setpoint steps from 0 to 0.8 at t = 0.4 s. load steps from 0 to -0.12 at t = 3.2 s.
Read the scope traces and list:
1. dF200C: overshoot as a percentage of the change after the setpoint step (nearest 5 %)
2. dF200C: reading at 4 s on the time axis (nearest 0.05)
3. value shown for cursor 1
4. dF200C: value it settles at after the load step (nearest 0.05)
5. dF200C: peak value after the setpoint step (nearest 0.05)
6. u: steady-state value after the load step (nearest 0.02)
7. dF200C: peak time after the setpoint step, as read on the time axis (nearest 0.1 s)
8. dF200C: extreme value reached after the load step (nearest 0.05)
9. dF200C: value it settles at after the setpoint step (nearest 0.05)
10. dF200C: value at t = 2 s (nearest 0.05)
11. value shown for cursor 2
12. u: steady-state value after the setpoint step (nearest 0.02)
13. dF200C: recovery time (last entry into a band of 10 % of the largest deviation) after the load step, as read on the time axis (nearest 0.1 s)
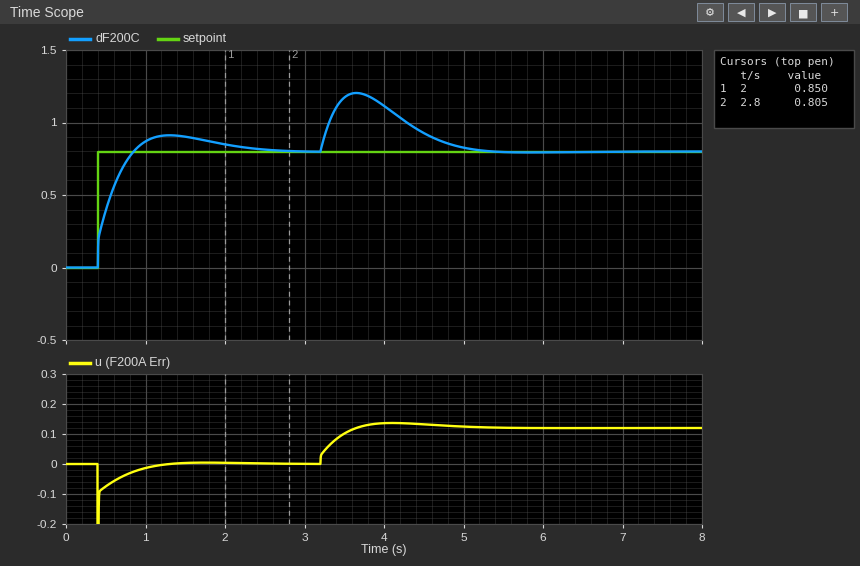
15 %
1.10
0.850
0.80
0.90
0.12
1.3 s
1.20
0.80
0.85
0.805
0.00
4.9 s
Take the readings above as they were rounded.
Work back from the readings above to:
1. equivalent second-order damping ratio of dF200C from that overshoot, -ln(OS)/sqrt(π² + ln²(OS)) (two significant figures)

0.52
